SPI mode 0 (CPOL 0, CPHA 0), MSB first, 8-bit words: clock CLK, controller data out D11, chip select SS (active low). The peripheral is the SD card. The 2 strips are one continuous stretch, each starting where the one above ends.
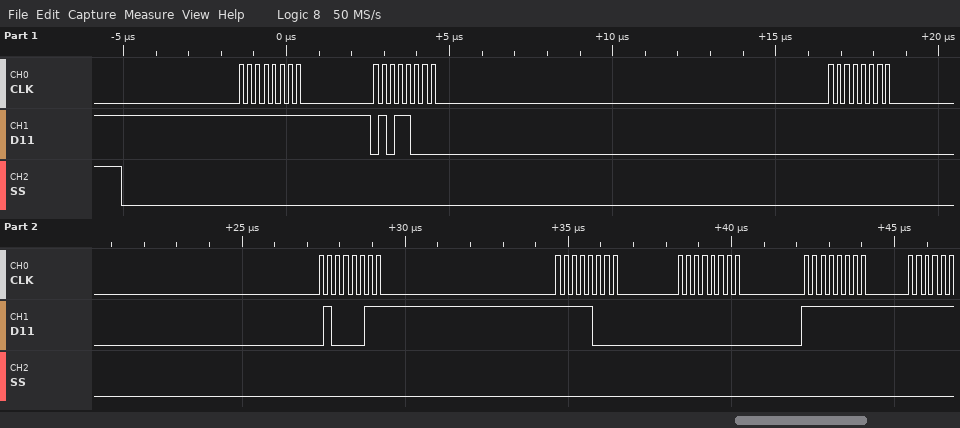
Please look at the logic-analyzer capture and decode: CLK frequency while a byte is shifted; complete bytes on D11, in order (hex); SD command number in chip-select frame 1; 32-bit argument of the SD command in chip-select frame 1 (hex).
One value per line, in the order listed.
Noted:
4 MHz
FF 58 00 43 F8 00 FF
CMD24
0x0043F800
